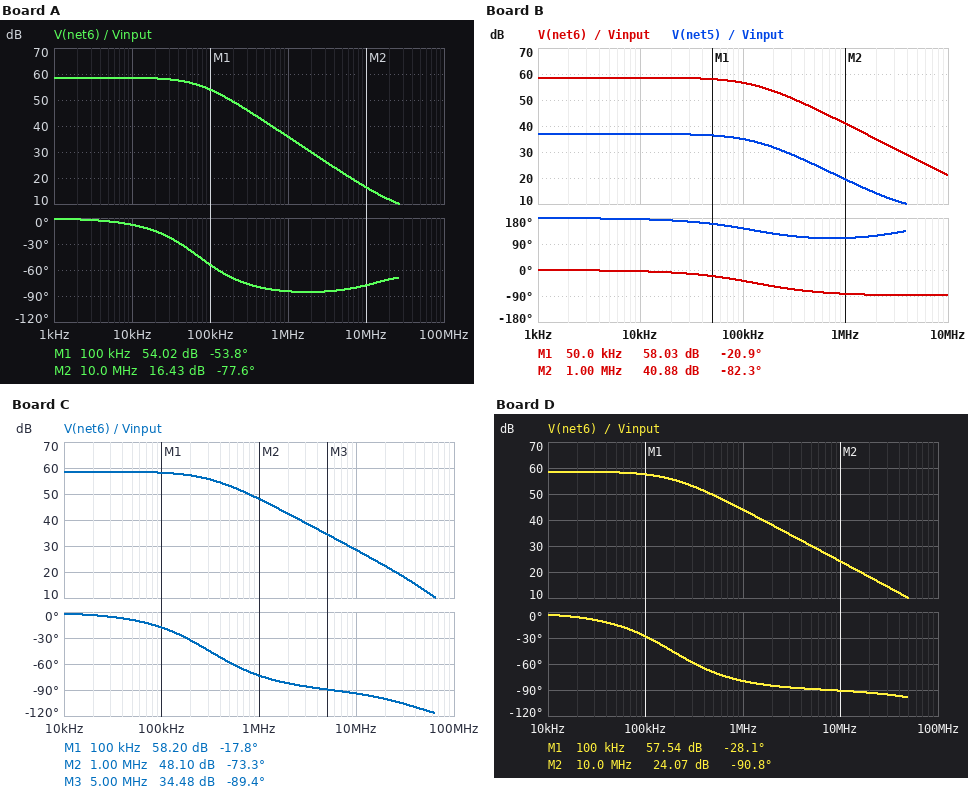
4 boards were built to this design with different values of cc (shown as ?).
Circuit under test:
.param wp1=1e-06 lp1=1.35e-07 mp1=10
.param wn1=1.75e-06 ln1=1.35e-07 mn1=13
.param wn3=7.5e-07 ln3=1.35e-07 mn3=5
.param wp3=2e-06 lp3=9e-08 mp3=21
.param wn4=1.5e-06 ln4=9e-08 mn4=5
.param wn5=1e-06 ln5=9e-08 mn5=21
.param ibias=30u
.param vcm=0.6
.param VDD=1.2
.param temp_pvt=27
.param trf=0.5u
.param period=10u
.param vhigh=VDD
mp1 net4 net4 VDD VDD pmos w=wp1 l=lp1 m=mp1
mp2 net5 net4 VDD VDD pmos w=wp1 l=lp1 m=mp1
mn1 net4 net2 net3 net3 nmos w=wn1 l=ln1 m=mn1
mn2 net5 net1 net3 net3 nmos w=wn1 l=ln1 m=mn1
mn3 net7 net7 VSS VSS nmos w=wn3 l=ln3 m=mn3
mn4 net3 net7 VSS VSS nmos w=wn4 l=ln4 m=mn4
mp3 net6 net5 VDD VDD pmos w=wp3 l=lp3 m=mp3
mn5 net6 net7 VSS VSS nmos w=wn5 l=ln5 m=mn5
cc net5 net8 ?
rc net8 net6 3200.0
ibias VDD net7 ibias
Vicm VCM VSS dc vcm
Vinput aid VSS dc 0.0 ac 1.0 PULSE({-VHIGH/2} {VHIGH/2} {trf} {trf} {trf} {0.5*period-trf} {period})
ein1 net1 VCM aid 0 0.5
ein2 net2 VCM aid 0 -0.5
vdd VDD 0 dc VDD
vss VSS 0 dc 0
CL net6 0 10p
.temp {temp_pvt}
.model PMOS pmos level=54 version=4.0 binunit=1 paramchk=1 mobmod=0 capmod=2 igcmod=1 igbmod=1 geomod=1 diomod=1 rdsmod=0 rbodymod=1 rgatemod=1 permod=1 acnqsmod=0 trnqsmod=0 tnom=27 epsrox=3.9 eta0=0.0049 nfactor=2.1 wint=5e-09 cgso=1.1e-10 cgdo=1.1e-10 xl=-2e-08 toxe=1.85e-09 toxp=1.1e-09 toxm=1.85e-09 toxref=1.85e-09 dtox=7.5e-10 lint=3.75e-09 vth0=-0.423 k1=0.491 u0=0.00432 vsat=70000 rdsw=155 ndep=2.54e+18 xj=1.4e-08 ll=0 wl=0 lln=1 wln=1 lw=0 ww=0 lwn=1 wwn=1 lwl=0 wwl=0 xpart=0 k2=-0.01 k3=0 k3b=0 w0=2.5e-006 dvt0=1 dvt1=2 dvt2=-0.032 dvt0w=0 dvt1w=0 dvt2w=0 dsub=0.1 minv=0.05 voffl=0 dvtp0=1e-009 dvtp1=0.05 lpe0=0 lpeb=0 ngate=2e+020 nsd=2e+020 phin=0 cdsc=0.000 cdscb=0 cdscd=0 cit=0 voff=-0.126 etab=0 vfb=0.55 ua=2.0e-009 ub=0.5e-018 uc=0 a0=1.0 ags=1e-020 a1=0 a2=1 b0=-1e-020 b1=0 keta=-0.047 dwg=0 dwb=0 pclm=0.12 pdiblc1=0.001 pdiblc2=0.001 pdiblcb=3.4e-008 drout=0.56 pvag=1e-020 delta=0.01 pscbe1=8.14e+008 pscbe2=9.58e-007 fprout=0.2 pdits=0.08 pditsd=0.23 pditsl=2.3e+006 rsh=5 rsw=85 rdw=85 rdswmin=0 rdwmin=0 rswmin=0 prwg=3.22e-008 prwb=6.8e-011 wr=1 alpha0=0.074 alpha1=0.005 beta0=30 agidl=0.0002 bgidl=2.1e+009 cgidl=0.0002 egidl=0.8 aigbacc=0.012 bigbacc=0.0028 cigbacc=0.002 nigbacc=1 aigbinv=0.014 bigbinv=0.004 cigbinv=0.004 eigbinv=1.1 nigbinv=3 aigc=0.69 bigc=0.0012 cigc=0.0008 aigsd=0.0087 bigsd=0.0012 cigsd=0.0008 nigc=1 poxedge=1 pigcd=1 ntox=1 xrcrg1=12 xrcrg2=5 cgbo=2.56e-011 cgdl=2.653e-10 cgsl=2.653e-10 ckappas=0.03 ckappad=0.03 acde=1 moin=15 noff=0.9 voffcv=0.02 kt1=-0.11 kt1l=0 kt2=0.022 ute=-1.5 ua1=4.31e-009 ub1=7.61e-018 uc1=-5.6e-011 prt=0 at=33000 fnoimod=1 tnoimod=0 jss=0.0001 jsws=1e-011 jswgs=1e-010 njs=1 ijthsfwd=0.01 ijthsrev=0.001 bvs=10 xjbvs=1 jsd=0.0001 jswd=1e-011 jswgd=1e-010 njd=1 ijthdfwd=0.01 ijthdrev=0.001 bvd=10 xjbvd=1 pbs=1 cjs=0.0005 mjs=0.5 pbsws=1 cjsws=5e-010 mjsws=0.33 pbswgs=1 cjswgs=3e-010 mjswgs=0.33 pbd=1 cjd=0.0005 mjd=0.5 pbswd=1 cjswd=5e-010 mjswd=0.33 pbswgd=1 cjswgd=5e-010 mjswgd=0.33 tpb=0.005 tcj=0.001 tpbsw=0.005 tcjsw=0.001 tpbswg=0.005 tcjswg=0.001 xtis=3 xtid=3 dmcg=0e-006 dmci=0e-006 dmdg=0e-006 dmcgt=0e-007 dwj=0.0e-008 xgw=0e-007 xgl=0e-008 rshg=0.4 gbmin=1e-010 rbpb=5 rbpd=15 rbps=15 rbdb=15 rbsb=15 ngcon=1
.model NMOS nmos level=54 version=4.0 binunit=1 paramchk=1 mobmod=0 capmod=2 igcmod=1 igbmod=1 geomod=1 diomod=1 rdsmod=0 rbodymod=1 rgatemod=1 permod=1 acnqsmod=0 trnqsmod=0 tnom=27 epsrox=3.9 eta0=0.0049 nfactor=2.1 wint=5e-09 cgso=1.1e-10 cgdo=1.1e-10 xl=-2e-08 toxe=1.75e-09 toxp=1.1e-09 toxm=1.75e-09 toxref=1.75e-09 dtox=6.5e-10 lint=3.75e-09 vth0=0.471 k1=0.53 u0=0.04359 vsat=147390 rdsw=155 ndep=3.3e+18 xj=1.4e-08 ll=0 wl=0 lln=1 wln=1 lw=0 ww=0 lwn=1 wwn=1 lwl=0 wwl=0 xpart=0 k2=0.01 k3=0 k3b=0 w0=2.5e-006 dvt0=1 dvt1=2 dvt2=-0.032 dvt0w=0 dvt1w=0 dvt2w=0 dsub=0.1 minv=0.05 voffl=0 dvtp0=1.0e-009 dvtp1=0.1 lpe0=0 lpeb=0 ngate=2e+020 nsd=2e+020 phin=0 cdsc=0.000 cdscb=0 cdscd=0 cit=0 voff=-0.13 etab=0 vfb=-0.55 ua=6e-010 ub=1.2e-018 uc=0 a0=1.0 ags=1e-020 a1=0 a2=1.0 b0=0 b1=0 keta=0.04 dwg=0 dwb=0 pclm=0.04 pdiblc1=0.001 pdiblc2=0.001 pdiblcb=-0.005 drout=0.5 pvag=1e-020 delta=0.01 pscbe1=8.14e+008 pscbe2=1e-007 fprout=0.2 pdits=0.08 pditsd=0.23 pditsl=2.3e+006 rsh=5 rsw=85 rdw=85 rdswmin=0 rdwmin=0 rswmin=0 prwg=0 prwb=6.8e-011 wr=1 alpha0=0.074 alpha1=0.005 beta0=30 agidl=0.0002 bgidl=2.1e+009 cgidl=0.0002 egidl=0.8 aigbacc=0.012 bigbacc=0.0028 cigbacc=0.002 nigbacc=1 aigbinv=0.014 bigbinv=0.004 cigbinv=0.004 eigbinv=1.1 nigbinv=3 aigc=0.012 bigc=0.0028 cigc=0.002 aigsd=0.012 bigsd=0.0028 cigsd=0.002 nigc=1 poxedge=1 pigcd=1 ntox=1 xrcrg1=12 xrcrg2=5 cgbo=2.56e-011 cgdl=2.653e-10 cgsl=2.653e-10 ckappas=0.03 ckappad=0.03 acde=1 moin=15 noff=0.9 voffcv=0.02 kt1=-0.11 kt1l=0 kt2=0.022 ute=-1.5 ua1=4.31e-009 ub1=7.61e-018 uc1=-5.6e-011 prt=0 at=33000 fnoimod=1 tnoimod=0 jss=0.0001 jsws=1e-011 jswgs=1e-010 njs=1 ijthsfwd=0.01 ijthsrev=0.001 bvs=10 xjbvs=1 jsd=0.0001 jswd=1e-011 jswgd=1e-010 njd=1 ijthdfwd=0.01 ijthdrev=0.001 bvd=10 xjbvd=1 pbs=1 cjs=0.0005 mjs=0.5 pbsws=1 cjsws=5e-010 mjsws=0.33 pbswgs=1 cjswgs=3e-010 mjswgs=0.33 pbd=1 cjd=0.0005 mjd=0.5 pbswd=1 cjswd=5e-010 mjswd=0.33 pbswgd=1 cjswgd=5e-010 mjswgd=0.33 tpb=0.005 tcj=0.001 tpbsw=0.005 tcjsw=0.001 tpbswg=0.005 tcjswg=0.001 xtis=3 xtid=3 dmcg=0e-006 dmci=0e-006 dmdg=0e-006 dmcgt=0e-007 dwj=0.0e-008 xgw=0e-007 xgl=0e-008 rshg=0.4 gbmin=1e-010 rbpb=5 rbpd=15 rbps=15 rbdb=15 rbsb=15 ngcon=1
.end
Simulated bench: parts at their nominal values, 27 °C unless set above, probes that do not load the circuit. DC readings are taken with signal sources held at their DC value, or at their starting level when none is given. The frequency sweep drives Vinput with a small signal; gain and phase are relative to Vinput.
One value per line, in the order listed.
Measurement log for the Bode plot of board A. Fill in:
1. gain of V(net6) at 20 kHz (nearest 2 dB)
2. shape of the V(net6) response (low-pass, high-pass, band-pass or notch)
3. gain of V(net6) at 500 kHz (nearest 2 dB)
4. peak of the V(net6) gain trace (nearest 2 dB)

58 dB
low-pass
42 dB
58 dB
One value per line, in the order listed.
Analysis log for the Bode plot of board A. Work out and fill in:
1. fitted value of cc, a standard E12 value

2.2 pF
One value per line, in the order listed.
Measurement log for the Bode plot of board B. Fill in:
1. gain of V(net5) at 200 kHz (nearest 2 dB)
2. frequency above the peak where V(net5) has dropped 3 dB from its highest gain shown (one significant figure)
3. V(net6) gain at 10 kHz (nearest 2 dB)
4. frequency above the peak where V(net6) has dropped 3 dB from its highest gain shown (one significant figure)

32 dB
100 kHz
58 dB
100 kHz
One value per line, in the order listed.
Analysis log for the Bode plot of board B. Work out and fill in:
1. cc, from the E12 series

1.2 pF
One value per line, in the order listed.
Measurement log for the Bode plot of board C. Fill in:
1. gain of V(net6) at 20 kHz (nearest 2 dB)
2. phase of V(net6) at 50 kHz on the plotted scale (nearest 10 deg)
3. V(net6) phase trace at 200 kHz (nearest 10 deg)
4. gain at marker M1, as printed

58 dB
-10 deg
-30 deg
58.20 dB
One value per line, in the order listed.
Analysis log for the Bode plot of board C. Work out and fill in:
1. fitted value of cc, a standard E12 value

470 fF
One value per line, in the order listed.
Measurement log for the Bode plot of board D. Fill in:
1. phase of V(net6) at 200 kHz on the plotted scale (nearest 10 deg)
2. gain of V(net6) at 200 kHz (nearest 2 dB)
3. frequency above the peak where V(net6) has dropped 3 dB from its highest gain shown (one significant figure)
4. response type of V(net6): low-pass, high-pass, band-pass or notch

-50 deg
56 dB
200 kHz
low-pass
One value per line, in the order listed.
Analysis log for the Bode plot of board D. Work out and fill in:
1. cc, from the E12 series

820 fF
